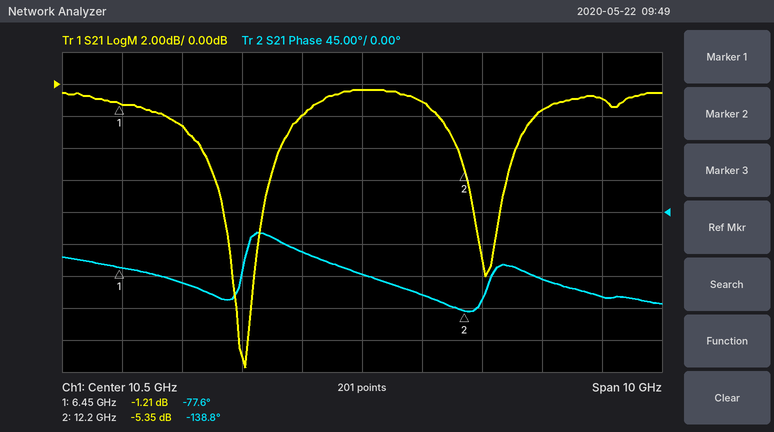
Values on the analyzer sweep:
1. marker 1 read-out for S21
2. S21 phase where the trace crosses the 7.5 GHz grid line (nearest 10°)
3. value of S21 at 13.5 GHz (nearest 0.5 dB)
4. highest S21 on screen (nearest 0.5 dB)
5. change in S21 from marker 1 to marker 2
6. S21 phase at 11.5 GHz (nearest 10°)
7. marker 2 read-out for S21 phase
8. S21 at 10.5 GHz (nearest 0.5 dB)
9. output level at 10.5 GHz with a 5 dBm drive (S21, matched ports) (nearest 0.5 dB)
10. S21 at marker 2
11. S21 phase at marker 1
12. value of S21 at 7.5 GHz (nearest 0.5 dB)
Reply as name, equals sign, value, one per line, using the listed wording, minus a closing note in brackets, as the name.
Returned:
marker 1 read-out for S21 = -1.21 dB
S21 phase where the trace crosses the 7.5 GHz grid line = -100°
value of S21 at 13.5 GHz = -1.5 dB
highest S21 on screen = -0.5 dB
change in S21 from marker 1 to marker 2 = -4.14 dB
S21 phase at 11.5 GHz = -120°
marker 2 read-out for S21 phase = -138.8°
S21 at 10.5 GHz = -0.5 dB
output level at 10.5 GHz with a 5 dBm drive (S21, matched ports) = 4.5 dBm
S21 at marker 2 = -5.35 dB
S21 phase at marker 1 = -77.6°
value of S21 at 7.5 GHz = -2.5 dB
